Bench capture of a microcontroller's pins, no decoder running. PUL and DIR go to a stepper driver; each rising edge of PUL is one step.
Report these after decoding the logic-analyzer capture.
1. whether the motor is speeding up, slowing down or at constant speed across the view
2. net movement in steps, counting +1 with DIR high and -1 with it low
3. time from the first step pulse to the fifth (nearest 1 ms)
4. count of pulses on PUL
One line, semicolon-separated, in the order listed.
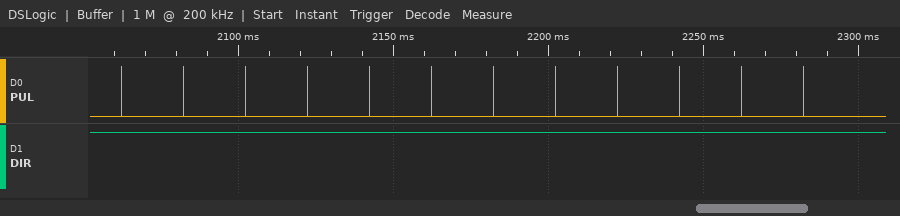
constant speed; +12; 80 ms; 12
